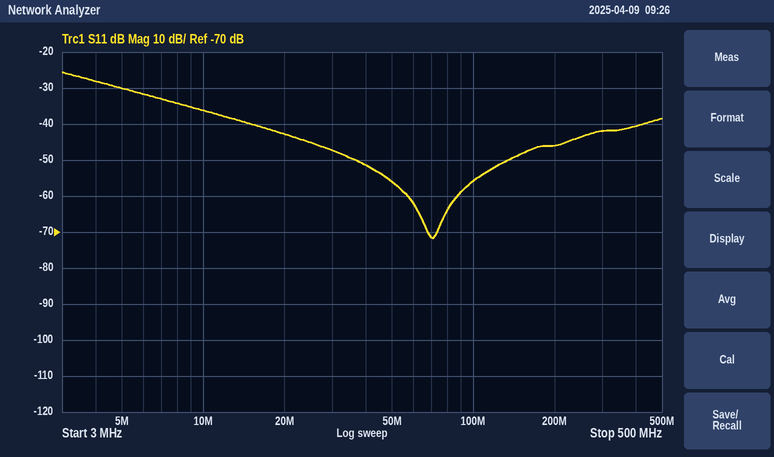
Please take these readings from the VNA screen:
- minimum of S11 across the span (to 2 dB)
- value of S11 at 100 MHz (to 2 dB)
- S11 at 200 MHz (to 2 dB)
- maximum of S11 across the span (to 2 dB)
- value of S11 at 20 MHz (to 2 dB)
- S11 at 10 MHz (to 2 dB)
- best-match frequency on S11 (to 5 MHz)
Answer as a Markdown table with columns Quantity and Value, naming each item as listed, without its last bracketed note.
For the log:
| Quantity | Value |
|---|---|
| minimum of S11 across the span | -72 dB |
| value of S11 at 100 MHz | -56 dB |
| S11 at 200 MHz | -46 dB |
| maximum of S11 across the span | -26 dB |
| value of S11 at 20 MHz | -42 dB |
| S11 at 10 MHz | -36 dB |
| best-match frequency on S11 | 70 MHz |
